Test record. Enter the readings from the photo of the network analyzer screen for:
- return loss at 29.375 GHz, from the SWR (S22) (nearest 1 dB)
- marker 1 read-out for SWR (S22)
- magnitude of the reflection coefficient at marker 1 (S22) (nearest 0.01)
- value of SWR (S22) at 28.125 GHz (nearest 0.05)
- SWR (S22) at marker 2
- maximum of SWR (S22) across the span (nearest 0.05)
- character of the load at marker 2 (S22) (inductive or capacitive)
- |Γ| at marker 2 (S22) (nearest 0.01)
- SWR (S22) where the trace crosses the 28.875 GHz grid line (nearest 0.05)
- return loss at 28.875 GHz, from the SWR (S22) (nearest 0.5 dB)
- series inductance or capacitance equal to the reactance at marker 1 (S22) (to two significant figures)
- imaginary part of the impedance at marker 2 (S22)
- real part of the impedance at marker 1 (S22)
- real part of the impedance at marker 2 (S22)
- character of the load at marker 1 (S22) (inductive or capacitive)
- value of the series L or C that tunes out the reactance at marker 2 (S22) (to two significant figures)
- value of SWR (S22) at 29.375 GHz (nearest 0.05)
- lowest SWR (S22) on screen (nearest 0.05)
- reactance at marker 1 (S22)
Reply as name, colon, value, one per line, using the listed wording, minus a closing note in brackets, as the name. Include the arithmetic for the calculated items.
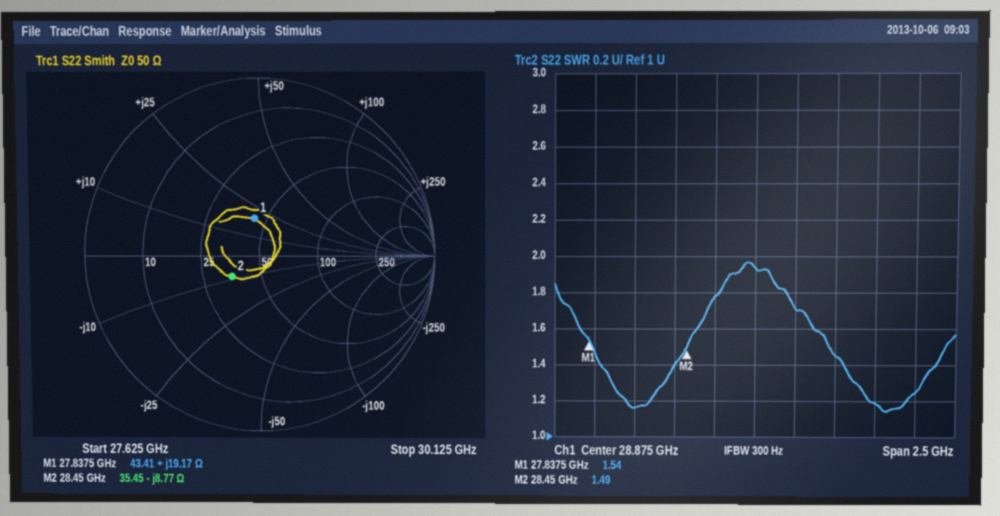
return loss at 29.375 GHz, from the SWR (S22): −20 log10((1.45 − 1)/(1.45 + 1)) ≈ 15 dB
marker 1 read-out for SWR: 1.54
magnitude of the reflection coefficient at marker 1 (S22): 0.21
value of SWR (S22) at 28.125 GHz: 1.15
SWR (S22) at marker 2: 1.49
maximum of SWR (S22) across the span: 1.95
character of the load at marker 2 (S22): capacitive
|Γ| at marker 2 (S22): 0.20
SWR (S22) where the trace crosses the 28.875 GHz grid line: 1.95
return loss at 28.875 GHz, from the SWR (S22): −20 log10((1.95 − 1)/(1.95 + 1)) ≈ 9.84 dB, so 10.0 dB to the nearest 0.5 dB
series inductance or capacitance equal to the reactance at marker 1 (S22): L = 19.17 Ω/(2π × 27.8375 GHz) ≈ 110 pH
imaginary part of the impedance at marker 2: -8.77 Ω
real part of the impedance at marker 1: 43.41 Ω
real part of the impedance at marker 2: 35.45 Ω
character of the load at marker 1 (S22): inductive
value of the series L or C that tunes out the reactance at marker 2 (S22): L = 8.77 Ω/(2π × 28.45 GHz) ≈ 49 pH
value of SWR (S22) at 29.375 GHz: 1.45
lowest SWR (S22) on screen: 1.15
reactance at marker 1: +19.17 Ω
